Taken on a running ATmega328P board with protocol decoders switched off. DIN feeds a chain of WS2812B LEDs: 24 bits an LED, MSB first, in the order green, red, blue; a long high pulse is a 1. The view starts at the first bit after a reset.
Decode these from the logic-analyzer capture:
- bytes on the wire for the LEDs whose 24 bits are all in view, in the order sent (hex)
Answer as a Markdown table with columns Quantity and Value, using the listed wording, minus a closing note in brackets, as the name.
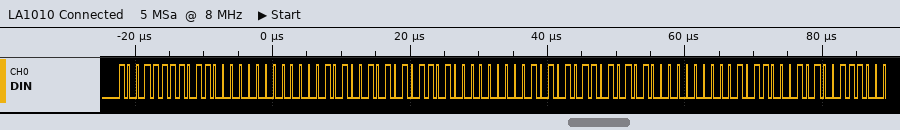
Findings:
| Quantity | Value |
|---|---|
| bytes on the wire for the LEDs whose 24 bits are all in view, in the order sent | 9F 60 00 A5 5A 00 AB 54 00 |
